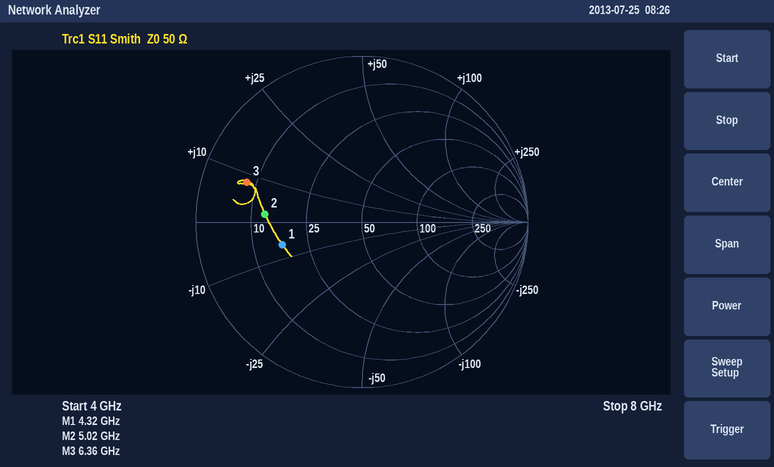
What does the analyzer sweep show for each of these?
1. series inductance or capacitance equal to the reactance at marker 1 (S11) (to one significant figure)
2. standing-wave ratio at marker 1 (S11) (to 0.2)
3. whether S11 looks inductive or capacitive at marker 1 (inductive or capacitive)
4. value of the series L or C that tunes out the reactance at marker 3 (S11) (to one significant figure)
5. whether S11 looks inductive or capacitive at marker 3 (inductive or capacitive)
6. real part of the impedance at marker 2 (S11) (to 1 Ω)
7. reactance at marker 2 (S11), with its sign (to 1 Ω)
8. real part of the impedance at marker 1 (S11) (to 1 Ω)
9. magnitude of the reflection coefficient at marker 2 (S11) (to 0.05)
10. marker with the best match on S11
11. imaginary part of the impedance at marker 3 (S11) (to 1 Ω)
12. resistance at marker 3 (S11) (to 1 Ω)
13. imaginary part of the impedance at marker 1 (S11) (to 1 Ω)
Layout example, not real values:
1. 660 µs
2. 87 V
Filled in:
1. 6 pF
2. 3.0
3. capacitive
4. 3 pF
5. inductive
6. 13 Ω
7. +2 Ω
8. 17 Ω
9. 0.60
10. marker 1
11. +8 Ω
12. 8 Ω
13. -6 Ω
